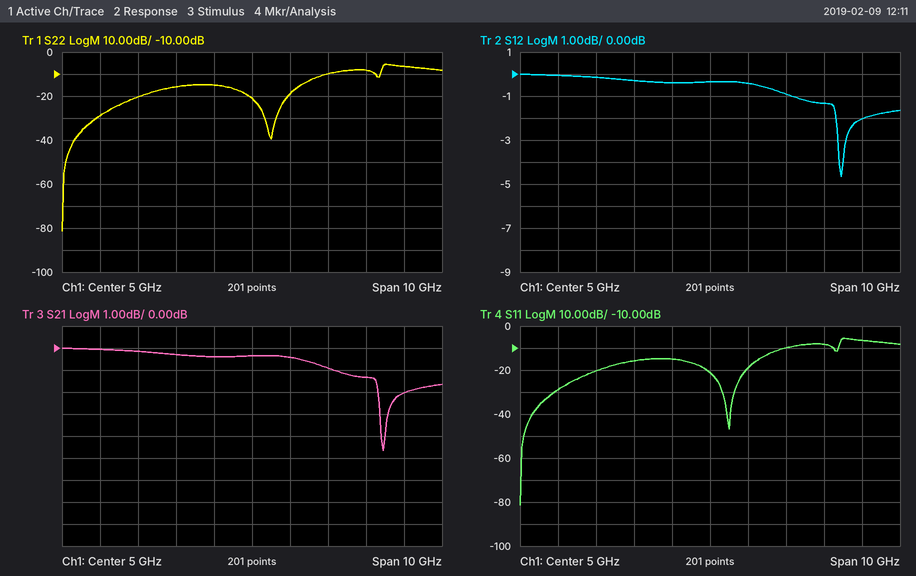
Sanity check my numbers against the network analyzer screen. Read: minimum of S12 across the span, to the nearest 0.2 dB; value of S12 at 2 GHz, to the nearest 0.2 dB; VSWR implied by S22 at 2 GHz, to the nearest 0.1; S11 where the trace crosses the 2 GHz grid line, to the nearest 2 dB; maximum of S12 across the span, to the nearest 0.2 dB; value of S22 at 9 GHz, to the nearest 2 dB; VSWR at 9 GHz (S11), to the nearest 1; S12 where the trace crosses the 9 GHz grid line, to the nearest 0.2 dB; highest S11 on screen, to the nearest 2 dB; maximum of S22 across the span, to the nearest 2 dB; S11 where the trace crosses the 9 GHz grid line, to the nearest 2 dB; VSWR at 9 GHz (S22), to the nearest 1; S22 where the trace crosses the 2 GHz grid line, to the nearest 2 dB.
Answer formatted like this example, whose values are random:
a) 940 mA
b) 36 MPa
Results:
a) -4.6 dB
b) -0.2 dB
c) 1.2
d) -20 dB
e) 0.0 dB
f) -6 dB
g) 3
h) -2.0 dB
i) -6 dB
j) -6 dB
k) -6 dB
l) 3
m) -20 dB
